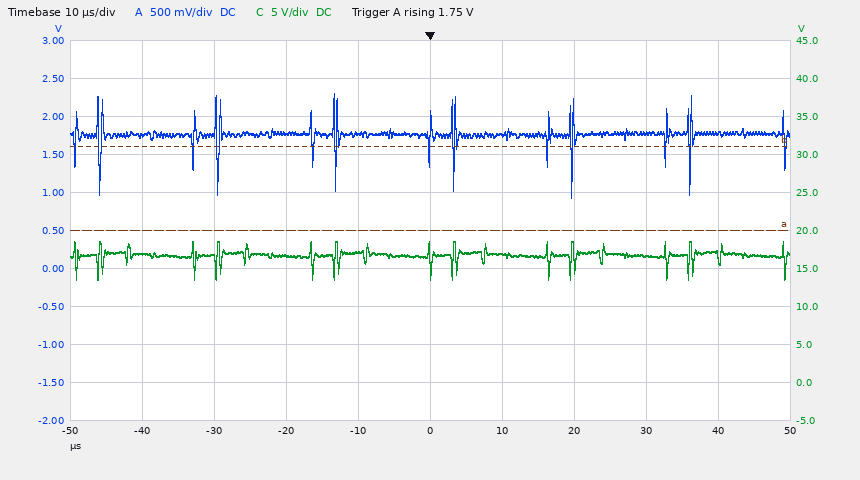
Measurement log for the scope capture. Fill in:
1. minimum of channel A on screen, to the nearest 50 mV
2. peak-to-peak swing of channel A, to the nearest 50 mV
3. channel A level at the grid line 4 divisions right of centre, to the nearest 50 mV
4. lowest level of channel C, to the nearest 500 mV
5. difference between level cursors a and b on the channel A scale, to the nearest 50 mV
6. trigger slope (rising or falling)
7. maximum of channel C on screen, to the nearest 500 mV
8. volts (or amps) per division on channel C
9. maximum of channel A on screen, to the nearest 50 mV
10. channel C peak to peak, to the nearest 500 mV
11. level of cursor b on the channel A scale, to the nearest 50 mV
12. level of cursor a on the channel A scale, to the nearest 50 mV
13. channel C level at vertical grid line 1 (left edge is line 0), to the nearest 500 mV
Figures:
950 mV
1.35 V
1.80 V
13.5 V
1.10 V
rising
18.5 V
5 V
2.30 V
5.0 V
1.60 V
500 mV
17.0 V
